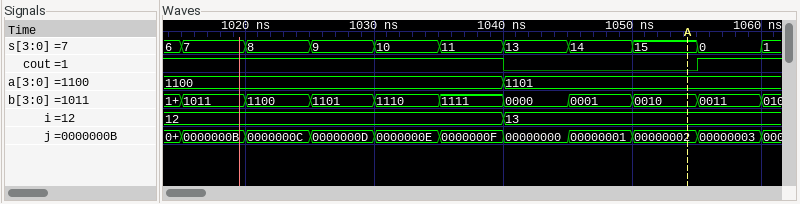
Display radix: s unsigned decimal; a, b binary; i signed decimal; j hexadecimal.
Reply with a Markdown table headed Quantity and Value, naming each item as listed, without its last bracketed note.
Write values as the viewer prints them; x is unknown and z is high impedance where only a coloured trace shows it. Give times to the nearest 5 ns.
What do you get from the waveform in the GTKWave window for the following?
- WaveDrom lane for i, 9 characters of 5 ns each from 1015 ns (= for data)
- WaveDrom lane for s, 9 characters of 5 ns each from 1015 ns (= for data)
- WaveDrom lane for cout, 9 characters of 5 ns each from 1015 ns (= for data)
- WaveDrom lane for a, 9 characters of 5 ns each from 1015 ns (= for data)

| Quantity | Value |
|---|---|
| WaveDrom lane for i, 9 characters of 5 ns each from 1015 ns | {name: 'i', wave: '=....=...', data: '12 13'} |
| WaveDrom lane for s, 9 characters of 5 ns each from 1015 ns | {name: 's', wave: '=========', data: '7 8 9 10 11 13 14 15 0'} |
| WaveDrom lane for cout, 9 characters of 5 ns each from 1015 ns | {name: 'cout', wave: '1....0..1'} |
| WaveDrom lane for a, 9 characters of 5 ns each from 1015 ns | {name: 'a', wave: '=....=...', data: '1100 1101'} |
